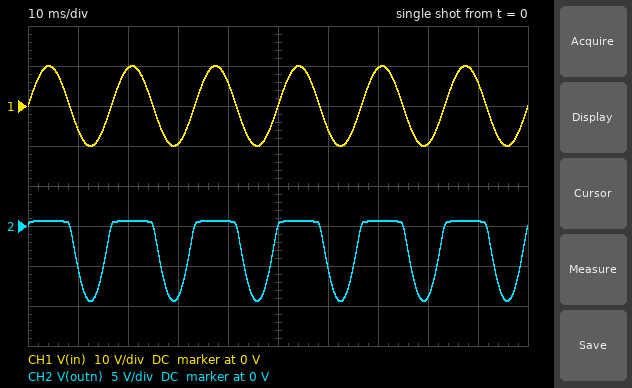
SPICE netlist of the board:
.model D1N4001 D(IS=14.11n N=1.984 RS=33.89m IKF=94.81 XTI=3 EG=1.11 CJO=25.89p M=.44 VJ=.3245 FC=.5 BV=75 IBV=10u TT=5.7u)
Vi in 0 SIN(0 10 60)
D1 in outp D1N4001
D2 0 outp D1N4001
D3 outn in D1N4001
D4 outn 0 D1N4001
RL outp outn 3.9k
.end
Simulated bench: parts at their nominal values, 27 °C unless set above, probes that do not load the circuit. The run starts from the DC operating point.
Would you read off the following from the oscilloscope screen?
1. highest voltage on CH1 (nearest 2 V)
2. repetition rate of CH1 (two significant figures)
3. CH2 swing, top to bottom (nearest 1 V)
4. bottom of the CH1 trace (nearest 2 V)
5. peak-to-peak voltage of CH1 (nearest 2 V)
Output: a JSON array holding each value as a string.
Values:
["10 V", "60 Hz", "10 V", "-10 V", "20 V"]
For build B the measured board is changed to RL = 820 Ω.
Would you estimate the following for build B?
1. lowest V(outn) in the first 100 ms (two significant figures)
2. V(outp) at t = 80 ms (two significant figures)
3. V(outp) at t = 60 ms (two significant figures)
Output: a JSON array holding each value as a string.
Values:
["-9.3 V", "-690 mV", "-660 mV"]
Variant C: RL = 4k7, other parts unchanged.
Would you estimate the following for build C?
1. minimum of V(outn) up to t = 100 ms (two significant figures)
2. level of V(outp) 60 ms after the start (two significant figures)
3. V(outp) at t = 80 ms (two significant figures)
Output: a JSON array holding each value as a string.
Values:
["-9.4 V", "-570 mV", "-600 mV"]
